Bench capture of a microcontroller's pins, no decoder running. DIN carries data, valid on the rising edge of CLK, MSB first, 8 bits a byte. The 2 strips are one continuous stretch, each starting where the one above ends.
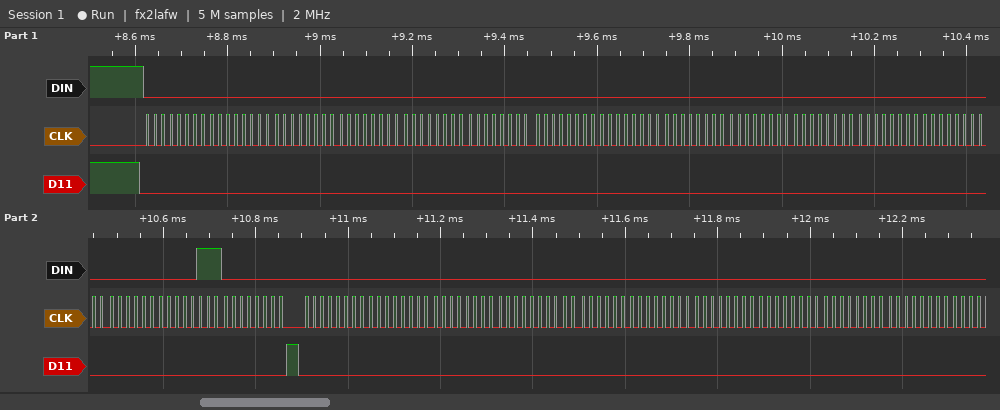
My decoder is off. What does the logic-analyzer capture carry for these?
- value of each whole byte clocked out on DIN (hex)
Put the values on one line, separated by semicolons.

00 00 00 00 00 00 00 00 00 00 00 00 00 00 07 00 00 00 00 00 00 00 00 00 00 00
